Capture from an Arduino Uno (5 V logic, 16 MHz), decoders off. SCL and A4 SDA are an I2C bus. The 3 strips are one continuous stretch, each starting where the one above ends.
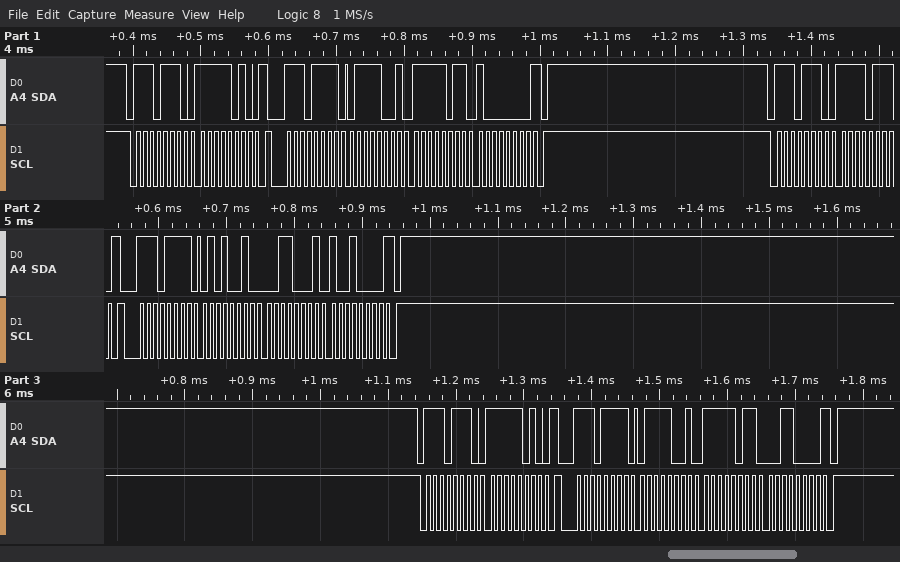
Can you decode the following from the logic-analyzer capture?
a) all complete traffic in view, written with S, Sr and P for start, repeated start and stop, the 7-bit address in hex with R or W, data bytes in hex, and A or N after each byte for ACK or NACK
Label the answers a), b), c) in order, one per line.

a) S 77W A FA A Sr 77R A 79 A FB A 80 N P S 77W A F7 A Sr 77R A 52 A 31 A 90 N P S 77W A FA A Sr 77R A 79 A FB A 30 N P
